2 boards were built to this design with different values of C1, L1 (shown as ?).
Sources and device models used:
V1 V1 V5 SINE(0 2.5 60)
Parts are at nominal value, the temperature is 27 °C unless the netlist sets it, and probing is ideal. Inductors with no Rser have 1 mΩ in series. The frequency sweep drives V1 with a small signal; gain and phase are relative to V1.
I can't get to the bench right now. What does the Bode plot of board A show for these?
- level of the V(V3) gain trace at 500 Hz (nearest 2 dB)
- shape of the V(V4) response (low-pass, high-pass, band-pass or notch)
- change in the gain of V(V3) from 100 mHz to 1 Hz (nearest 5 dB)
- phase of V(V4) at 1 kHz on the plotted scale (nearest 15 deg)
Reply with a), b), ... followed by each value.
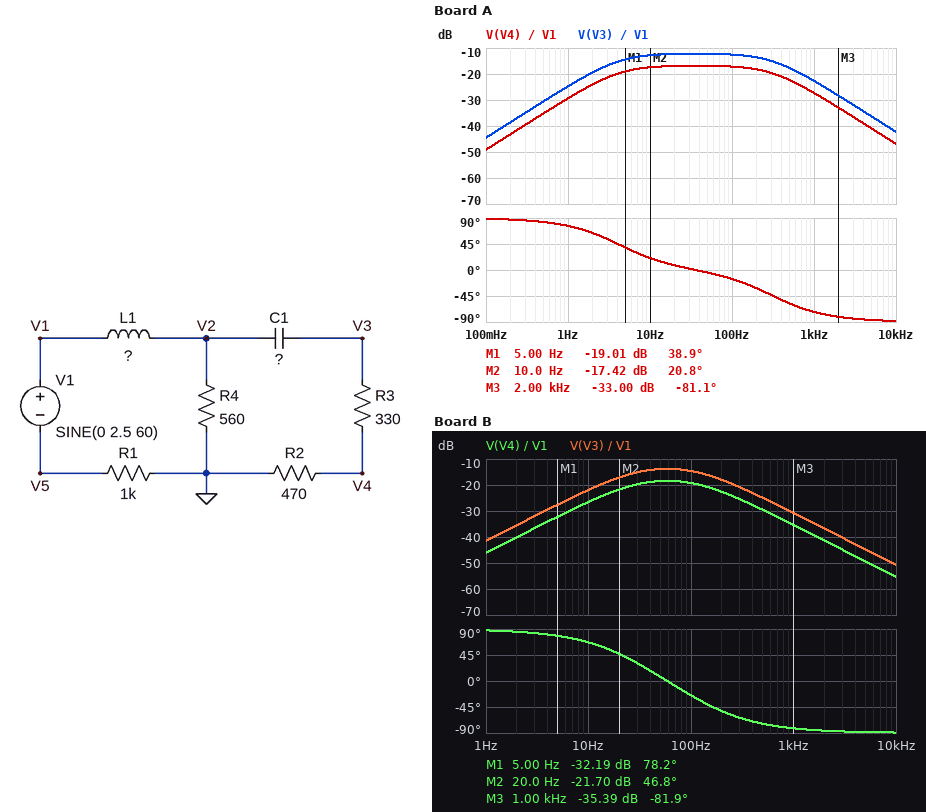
a) -18 dB
b) band-pass
c) 20 dB
d) -75 deg
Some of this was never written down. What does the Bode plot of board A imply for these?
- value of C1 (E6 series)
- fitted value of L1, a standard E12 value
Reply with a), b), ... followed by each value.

a) 33 µF
b) 680 mH
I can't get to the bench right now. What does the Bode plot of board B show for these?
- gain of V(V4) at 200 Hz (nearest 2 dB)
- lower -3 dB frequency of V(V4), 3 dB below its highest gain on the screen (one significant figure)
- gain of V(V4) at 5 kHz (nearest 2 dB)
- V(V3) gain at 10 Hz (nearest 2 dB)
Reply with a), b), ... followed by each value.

a) -22 dB
b) 20 Hz
c) -50 dB
d) -22 dB
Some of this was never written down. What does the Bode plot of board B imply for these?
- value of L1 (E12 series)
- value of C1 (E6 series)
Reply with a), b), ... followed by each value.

a) 1.8 H
b) 4.7 µF
